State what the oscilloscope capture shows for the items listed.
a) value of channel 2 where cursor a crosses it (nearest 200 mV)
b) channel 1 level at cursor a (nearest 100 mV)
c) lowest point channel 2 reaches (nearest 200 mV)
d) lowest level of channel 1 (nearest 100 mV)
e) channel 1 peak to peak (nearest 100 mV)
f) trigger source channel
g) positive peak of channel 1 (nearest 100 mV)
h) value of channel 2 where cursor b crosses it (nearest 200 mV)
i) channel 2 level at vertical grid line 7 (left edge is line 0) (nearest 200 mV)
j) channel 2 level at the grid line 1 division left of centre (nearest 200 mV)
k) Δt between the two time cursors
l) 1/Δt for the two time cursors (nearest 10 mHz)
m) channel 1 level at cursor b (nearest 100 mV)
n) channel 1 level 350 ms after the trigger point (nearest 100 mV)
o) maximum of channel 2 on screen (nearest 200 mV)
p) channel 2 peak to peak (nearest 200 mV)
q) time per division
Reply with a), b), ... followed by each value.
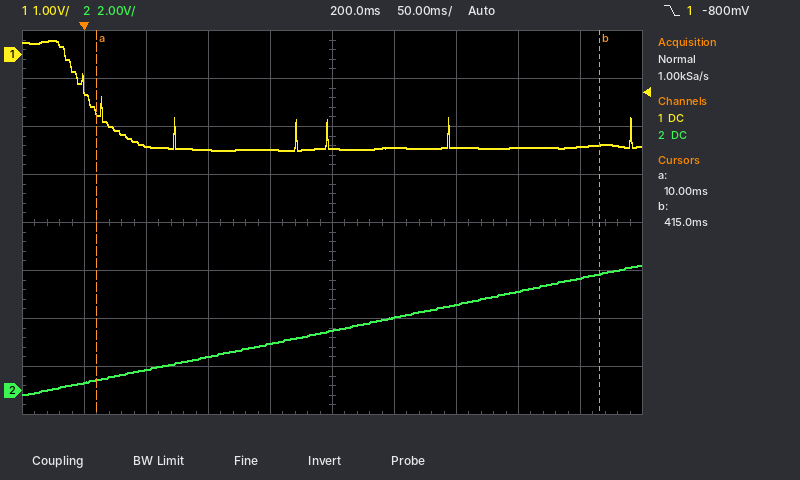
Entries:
a) 400 mV
b) -1.2 V
c) -200 mV
d) -2.0 V
e) 2.3 V
f) channel 1
g) 300 mV
h) 4.8 V
i) 3.6 V
j) 2.0 V
k) 405 ms
l) 2.47 Hz
m) -1.9 V
n) -1.9 V
o) 5.2 V
p) 5.4 V
q) 50 ms
